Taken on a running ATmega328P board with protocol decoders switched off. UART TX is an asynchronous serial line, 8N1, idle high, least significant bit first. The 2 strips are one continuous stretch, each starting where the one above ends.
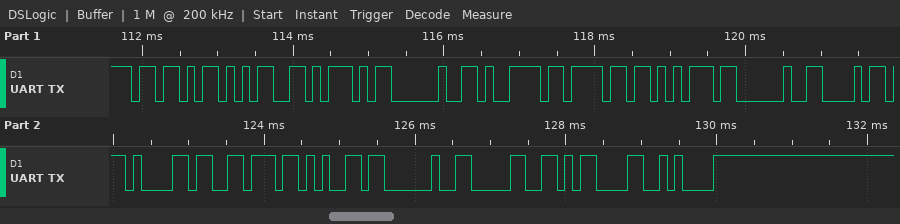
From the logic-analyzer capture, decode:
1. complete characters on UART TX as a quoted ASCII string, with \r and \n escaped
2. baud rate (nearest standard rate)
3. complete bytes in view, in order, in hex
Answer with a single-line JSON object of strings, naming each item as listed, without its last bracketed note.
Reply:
{"complete characters on UART TX as a quoted ASCII string, with \\r and \\n escaped": "\"[5] you have 0\\r\\n\"", "baud rate": "9600 baud", "complete bytes in view, in order, in hex": "5B 35 5D 20 79 6F 75 20 68 61 76 65 20 30 0D 0A"}
